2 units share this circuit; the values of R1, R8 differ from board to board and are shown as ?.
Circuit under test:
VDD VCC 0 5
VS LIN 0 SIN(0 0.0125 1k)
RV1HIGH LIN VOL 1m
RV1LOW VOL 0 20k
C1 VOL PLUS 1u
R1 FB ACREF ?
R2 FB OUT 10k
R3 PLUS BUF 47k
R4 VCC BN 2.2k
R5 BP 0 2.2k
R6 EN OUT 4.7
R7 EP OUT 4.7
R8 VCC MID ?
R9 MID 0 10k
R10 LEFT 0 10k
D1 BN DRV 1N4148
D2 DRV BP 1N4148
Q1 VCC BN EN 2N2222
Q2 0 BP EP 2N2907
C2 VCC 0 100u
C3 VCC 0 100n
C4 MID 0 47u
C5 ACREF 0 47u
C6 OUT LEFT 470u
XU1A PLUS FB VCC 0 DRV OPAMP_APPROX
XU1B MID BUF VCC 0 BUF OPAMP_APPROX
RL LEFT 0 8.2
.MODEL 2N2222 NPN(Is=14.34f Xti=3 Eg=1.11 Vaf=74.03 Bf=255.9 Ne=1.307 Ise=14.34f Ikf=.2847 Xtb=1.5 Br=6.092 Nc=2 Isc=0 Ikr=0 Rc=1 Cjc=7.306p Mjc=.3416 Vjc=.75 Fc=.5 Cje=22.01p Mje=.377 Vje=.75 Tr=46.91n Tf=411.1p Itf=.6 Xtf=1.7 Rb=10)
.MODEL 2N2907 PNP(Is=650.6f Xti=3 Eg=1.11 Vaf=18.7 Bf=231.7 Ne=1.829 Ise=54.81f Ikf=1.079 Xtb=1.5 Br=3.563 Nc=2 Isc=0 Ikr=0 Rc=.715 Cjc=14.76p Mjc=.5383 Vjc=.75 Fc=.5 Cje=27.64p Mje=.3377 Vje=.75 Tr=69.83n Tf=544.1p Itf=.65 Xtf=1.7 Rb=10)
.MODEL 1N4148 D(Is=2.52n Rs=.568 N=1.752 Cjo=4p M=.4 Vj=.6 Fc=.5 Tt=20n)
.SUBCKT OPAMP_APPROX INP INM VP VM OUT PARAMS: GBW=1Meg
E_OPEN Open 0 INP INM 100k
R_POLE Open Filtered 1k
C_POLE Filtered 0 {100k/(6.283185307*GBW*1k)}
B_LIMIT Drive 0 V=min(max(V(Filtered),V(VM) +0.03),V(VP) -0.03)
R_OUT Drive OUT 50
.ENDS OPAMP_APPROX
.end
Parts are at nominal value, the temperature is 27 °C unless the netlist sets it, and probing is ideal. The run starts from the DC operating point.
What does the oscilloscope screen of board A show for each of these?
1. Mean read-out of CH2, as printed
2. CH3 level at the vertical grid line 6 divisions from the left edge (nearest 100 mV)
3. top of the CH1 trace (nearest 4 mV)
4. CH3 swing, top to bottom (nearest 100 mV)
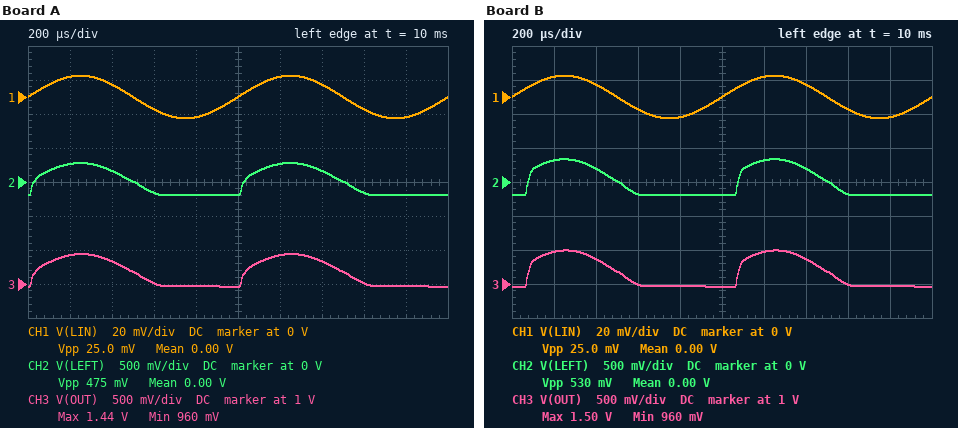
0.00 V
1.4 V
12 mV
500 mV
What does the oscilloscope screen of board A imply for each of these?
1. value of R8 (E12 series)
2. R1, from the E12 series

33 kΩ
470 Ω
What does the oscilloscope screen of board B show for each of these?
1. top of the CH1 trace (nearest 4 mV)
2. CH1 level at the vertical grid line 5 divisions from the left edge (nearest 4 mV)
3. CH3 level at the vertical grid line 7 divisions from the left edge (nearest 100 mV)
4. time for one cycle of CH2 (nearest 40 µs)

12 mV
0 V
1.4 V
1.00 ms
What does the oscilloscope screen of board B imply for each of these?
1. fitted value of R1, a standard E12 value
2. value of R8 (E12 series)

390 Ω
33 kΩ
